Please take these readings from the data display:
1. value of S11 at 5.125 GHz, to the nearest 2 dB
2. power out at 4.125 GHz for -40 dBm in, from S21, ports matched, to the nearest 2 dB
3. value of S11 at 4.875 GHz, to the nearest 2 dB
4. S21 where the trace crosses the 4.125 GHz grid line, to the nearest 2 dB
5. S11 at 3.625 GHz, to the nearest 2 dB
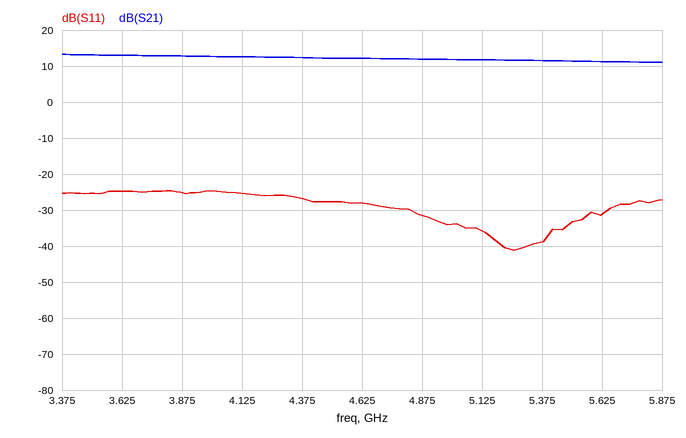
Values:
-36 dB
-28 dBm
-32 dB
12 dB
-24 dB
